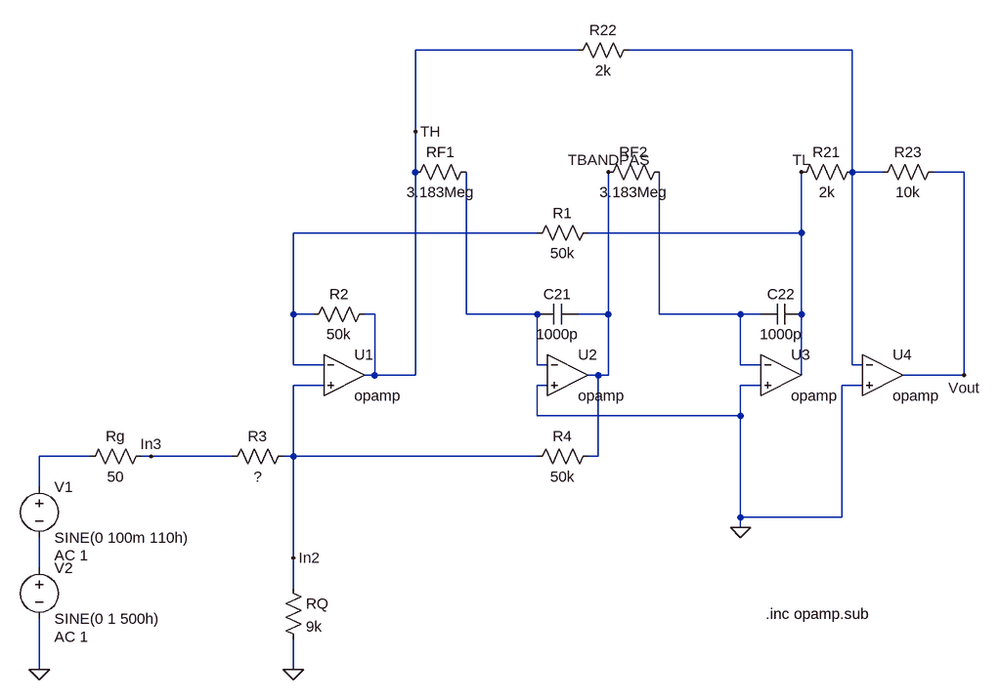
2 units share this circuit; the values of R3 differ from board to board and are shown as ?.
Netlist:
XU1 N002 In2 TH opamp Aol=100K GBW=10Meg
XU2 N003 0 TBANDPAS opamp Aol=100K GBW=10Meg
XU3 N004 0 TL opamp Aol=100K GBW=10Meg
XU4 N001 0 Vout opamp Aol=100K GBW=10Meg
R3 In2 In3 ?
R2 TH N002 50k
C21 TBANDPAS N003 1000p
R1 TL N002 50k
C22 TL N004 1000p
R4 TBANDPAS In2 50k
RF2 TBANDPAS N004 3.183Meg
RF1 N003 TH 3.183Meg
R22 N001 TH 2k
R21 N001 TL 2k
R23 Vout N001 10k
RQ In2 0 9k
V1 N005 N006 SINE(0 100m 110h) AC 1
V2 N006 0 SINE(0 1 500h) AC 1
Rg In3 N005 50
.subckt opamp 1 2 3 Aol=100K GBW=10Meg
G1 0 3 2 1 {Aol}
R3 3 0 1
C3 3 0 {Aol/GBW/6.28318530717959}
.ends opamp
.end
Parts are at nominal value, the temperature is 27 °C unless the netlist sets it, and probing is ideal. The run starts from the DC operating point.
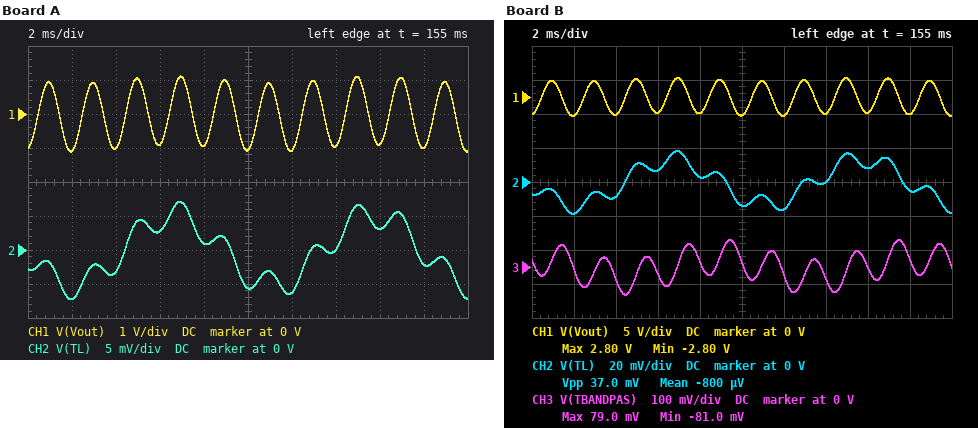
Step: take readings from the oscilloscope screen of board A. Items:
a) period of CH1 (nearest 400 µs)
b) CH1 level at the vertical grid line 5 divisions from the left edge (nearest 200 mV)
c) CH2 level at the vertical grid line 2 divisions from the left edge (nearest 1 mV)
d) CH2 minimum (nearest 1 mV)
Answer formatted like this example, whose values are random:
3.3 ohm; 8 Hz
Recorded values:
2.0 ms; -1.0 V; -3 mV; -7 mV
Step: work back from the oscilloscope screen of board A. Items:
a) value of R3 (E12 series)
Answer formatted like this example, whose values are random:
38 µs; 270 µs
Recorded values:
68 kΩ
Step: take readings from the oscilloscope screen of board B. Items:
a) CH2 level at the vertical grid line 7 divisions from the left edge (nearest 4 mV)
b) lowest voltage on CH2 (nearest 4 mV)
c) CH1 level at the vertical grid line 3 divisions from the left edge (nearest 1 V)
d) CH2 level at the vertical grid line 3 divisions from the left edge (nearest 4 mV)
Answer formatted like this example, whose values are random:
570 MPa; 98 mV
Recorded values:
0 V; -20 mV; -2 V; 8 mV
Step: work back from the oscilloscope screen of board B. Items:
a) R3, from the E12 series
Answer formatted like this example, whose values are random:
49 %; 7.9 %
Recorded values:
22 kΩ
